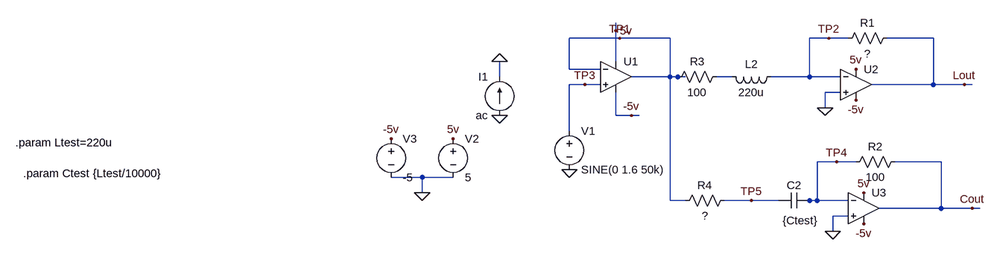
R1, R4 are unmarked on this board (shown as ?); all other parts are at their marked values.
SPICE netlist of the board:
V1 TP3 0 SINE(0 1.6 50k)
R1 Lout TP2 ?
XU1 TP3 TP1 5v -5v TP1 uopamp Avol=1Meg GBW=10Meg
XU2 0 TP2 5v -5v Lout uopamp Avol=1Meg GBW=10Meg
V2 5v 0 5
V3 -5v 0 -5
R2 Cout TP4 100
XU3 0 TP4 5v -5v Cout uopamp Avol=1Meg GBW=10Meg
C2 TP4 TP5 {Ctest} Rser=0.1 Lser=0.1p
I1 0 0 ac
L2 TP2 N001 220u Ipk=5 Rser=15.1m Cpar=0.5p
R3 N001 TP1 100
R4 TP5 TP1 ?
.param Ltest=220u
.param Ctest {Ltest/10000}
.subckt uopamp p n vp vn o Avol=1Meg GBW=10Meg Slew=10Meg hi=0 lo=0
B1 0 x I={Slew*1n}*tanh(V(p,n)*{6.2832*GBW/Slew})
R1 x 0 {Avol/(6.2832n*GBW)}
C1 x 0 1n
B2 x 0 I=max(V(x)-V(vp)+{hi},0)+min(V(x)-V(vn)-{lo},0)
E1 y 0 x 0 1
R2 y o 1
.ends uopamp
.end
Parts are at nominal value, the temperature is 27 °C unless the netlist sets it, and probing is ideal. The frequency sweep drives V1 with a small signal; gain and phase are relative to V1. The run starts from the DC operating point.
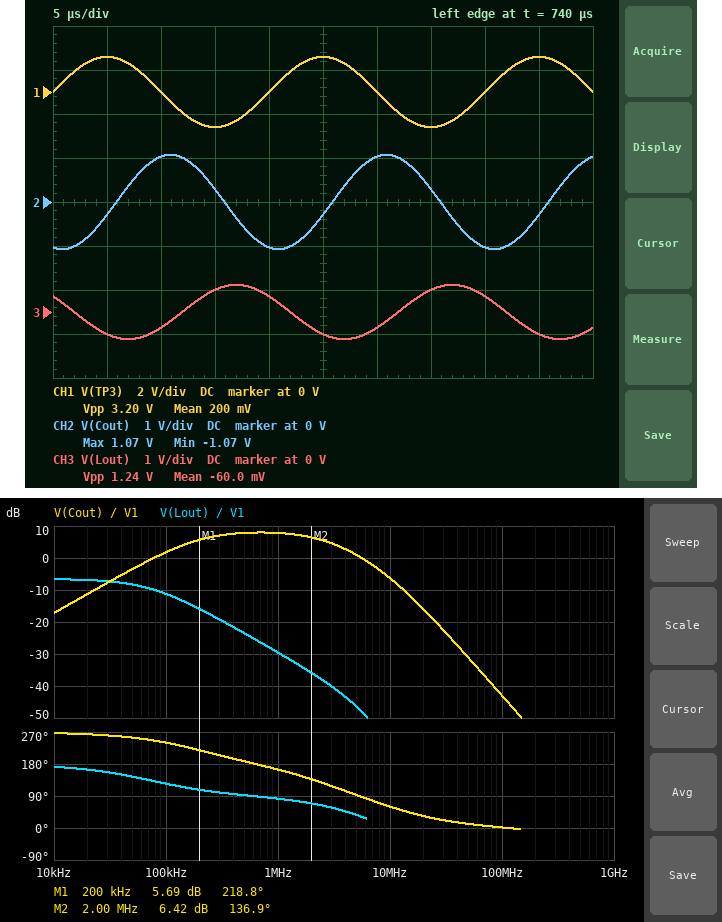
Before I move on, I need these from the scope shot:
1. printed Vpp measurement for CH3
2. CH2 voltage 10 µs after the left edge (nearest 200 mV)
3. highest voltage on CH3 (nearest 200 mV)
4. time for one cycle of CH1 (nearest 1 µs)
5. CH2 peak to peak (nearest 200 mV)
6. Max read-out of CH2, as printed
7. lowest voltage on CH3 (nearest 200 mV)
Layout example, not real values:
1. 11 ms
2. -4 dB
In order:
1. 1.24 V
2. 1.0 V
3. 600 mV
4. 20 µs
5. 2.2 V
6. 1.07 V
7. -600 mV
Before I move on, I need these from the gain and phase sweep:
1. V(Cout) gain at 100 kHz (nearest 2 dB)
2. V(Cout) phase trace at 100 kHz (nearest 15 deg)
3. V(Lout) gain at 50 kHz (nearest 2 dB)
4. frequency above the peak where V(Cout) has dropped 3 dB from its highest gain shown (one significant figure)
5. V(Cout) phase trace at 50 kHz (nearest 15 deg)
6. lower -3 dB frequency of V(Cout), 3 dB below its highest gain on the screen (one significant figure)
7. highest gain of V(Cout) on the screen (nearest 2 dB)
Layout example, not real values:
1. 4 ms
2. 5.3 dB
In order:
1. 2 dB
2. 240 deg
3. -8 dB
4. 3 MHz
5. 255 deg
6. 200 kHz
7. 8 dB
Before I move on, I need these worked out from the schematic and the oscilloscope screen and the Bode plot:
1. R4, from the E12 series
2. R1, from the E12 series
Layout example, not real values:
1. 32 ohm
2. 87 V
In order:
1. 39 Ω
2. 47 Ω
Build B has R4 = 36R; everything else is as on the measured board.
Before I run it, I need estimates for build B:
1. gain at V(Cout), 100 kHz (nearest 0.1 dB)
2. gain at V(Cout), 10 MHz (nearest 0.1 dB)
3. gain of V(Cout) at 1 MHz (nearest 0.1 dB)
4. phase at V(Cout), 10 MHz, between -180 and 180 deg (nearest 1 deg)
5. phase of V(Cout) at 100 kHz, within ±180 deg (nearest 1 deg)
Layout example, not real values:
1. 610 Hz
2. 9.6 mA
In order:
1. 1.9 dB
2. -6.1 dB
3. 8.5 dB
4. 59 deg
5. -118 deg
